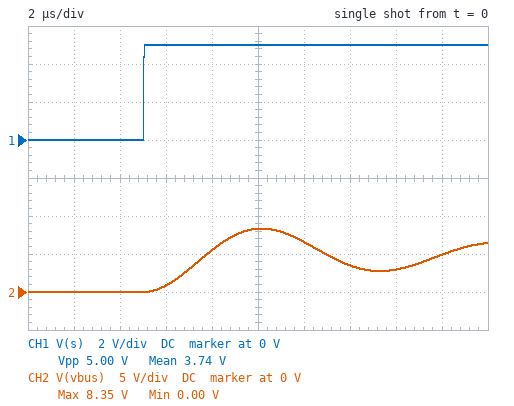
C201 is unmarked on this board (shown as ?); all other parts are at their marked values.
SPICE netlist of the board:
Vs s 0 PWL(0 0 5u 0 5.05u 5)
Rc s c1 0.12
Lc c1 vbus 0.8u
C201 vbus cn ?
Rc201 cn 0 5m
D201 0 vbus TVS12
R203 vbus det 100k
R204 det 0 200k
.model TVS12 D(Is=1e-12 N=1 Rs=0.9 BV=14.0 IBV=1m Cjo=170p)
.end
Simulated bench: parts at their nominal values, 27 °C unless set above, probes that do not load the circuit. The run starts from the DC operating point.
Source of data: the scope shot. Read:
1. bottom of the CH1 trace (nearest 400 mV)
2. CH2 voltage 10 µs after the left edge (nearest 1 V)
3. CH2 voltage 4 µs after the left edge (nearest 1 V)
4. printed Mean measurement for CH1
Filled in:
0 V
8 V
0 V
3.74 V
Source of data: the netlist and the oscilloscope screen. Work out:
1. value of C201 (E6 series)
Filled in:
3.3 µF
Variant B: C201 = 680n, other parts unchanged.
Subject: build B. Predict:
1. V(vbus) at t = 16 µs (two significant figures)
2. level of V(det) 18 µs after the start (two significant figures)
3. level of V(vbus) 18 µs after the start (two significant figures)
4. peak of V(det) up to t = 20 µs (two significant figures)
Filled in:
6.3 V
3.1 V
4.6 V
6.1 V
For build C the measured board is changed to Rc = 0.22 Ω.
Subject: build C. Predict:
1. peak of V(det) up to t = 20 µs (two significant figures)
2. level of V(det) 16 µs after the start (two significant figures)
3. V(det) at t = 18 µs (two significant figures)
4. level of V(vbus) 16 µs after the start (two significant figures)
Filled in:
4.9 V
2.6 V
3.2 V
3.9 V
